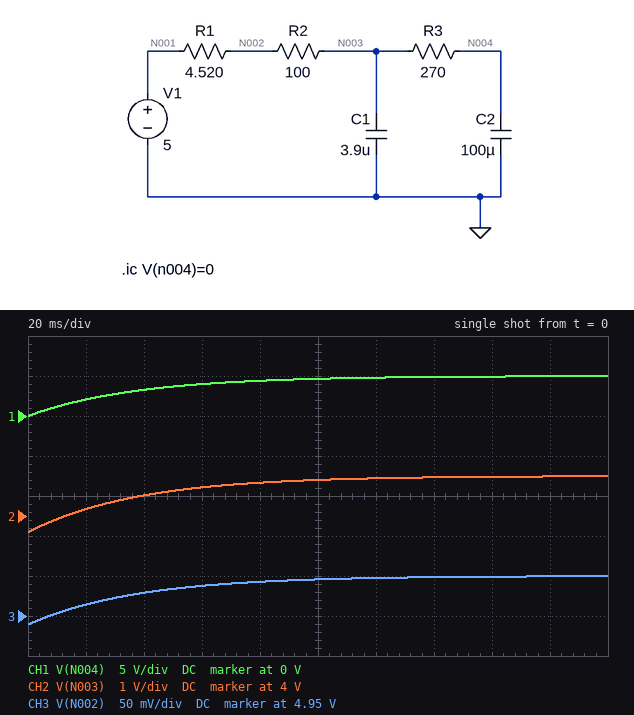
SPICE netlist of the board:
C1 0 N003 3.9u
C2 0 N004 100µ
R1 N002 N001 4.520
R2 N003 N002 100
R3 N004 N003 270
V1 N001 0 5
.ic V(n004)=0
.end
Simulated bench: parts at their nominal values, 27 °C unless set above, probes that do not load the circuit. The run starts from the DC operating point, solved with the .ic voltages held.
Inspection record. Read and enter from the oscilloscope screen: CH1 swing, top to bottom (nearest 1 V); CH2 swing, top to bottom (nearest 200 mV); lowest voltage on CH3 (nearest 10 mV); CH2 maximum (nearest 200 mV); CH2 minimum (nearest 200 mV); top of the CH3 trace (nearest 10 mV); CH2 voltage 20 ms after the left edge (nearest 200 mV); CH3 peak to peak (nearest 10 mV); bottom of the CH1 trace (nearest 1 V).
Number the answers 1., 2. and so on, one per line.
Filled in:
1. 5 V
2. 1.4 V
3. 4.94 V
4. 5.0 V
5. 3.6 V
6. 5.00 V
7. 4.2 V
8. 60 mV
9. 0 V
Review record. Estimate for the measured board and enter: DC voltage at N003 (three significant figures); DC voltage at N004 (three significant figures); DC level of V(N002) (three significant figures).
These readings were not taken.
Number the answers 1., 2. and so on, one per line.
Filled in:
1. 5.00 V
2. 5.00 V
3. 5.00 V
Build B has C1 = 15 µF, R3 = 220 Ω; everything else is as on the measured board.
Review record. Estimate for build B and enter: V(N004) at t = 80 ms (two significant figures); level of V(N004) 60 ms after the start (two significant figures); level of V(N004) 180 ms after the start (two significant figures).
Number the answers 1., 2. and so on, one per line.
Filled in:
1. 4.6 V
2. 4.2 V
3. 5.0 V
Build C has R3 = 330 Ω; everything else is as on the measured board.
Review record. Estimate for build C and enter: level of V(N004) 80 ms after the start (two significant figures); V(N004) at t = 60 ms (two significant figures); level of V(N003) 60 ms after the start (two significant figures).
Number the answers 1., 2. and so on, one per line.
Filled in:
1. 4.2 V
2. 3.7 V
3. 4.7 V
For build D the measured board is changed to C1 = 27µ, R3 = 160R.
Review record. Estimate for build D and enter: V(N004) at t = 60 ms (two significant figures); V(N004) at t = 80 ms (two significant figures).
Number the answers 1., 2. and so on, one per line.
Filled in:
1. 4.4 V
2. 4.7 V
